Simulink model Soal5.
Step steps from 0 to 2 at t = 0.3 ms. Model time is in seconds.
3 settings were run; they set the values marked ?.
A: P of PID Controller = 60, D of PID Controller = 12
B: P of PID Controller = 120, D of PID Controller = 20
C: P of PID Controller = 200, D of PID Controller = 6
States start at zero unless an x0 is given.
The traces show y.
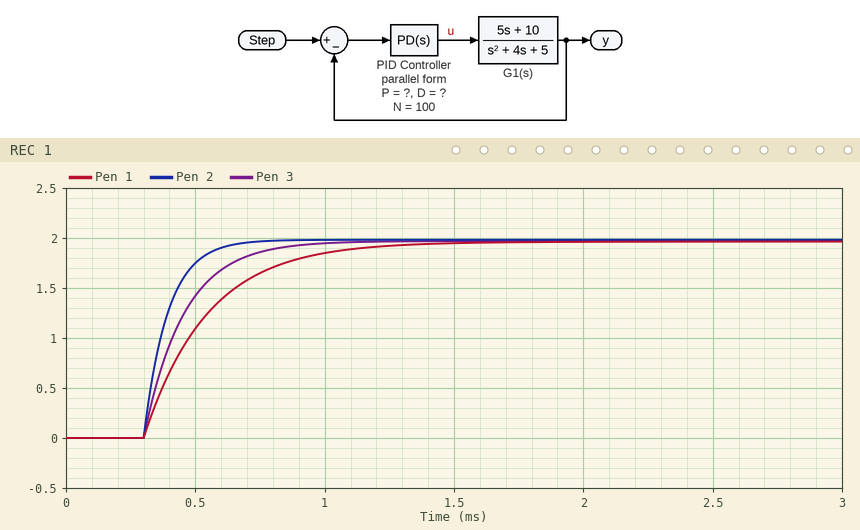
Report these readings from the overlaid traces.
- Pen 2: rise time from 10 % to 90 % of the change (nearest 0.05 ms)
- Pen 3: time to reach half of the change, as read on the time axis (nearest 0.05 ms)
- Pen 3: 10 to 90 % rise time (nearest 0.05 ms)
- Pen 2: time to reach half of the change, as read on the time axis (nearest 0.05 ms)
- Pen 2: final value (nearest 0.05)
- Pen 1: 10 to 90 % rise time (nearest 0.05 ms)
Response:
0.20 ms
0.40 ms
0.35 ms
0.35 ms
2.00
0.55 ms
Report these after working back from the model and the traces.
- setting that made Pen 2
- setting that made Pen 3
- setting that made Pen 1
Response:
B
A
C
